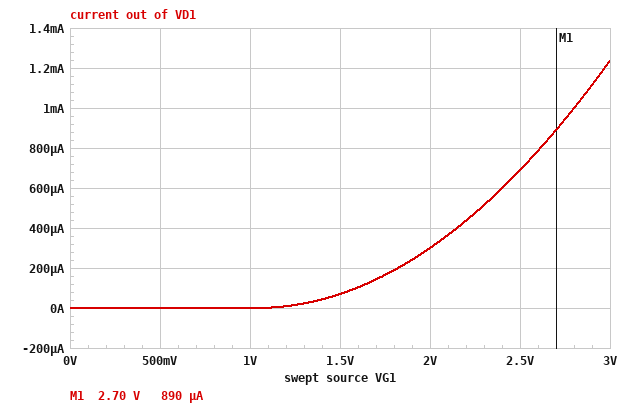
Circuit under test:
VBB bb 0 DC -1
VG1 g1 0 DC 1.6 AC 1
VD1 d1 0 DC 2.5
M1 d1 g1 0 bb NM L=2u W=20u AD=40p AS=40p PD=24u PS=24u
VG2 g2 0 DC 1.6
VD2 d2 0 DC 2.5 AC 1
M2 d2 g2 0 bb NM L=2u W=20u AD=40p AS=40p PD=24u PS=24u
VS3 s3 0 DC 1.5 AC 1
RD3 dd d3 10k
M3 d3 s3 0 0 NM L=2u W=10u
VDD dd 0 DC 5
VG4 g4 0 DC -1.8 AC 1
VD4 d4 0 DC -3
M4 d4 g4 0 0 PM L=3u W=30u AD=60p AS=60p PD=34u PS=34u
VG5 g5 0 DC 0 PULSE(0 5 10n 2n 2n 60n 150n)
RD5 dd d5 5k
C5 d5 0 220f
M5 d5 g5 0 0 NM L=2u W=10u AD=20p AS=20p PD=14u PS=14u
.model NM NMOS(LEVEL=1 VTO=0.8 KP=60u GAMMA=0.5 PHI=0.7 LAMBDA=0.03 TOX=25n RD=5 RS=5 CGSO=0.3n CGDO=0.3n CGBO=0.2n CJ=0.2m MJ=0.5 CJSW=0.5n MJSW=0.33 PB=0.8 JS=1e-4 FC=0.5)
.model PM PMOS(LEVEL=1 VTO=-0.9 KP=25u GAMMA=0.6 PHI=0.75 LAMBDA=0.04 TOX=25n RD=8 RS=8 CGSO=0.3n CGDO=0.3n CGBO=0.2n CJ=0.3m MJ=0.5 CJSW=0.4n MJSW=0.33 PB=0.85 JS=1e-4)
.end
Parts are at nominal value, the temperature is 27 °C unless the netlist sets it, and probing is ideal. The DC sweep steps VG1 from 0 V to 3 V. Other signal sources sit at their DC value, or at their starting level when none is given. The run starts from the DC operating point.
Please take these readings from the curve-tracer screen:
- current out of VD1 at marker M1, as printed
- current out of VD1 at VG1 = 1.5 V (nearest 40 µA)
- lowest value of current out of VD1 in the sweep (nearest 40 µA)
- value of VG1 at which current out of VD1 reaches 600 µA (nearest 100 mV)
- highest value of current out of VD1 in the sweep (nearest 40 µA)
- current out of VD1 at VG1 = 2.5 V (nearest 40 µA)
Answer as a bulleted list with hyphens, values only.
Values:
- 890 µA
- 80 µA
- 0 A
- 2.4 V
- 1.24 mA
- 680 µA
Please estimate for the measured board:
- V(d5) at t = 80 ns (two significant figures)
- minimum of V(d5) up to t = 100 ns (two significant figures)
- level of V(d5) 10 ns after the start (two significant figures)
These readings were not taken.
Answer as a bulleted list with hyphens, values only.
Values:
- 5.0 V
- 730 mV
- 5.0 V
